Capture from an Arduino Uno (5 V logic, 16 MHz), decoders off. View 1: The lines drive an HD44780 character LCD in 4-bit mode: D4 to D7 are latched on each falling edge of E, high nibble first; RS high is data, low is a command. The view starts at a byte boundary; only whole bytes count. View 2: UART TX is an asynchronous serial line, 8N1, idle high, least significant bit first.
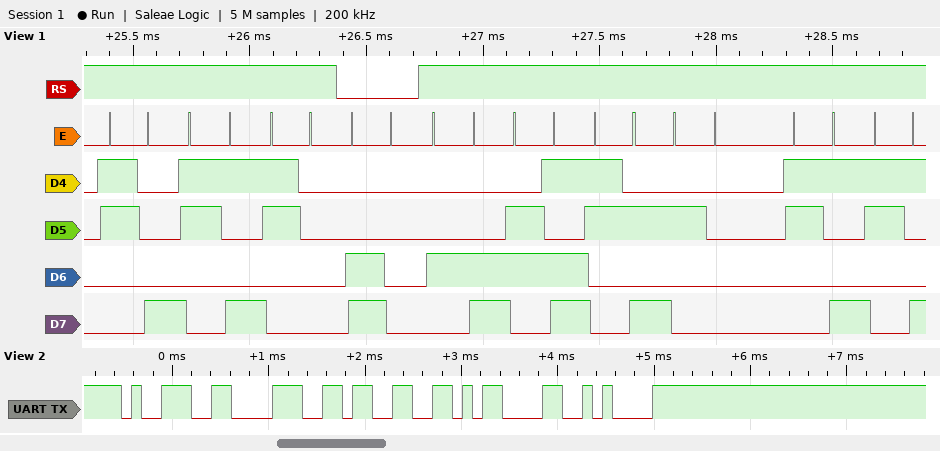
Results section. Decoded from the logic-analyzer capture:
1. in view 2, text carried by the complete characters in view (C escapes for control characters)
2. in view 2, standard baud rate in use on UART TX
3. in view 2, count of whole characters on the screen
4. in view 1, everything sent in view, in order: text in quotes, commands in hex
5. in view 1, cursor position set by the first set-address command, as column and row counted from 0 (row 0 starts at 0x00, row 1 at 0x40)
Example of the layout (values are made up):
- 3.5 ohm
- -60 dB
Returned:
- "983\r\n"
- 9600 baud
- 5
- "890" 0xC0 "Lm: 99"
- column 0, row 1
